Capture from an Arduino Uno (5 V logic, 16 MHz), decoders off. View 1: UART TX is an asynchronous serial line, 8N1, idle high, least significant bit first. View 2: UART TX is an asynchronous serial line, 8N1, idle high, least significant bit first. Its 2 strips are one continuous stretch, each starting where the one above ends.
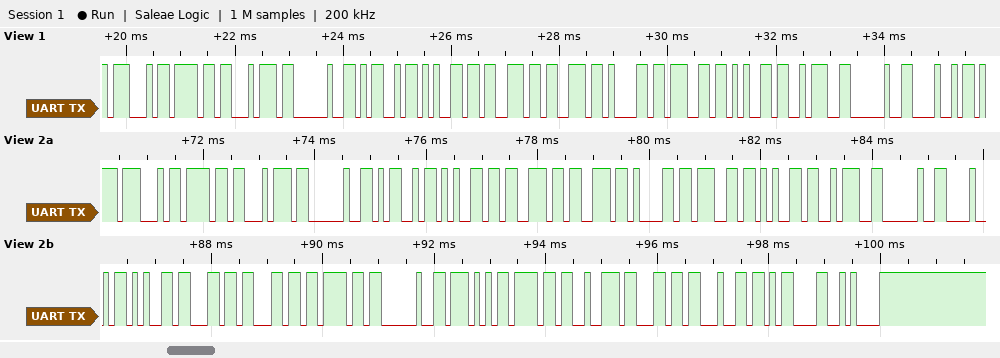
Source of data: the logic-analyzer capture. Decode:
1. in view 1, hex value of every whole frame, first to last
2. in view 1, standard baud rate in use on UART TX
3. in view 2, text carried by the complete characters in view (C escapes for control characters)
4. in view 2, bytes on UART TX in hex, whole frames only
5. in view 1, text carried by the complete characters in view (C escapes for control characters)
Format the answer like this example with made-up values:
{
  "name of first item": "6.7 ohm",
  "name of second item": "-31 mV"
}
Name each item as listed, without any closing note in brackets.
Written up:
{
  "in view 1, hex value of every whole frame, first to last": "0x47 0x6F 0x74 0x20 0x4D 0x65 0x73 0x73 0x61 0x67 0x65 0x3A 0x20 0x48",
  "in view 1, standard baud rate in use on UART TX": "9600 baud",
  "in view 2, text carried by the complete characters in view": "\"Got Message: Hello World\\r\\n\"",
  "in view 2, bytes on UART TX in hex, whole frames only": "0x47 0x6F 0x74 0x20 0x4D 0x65 0x73 0x73 0x61 0x67 0x65 0x3A 0x20 0x48 0x65 0x6C 0x6C 0x6F 0x20 0x57 0x6F 0x72 0x6C 0x64 0x0D 0x0A",
  "in view 1, text carried by the complete characters in view": "\"Got Message: H\""
}
